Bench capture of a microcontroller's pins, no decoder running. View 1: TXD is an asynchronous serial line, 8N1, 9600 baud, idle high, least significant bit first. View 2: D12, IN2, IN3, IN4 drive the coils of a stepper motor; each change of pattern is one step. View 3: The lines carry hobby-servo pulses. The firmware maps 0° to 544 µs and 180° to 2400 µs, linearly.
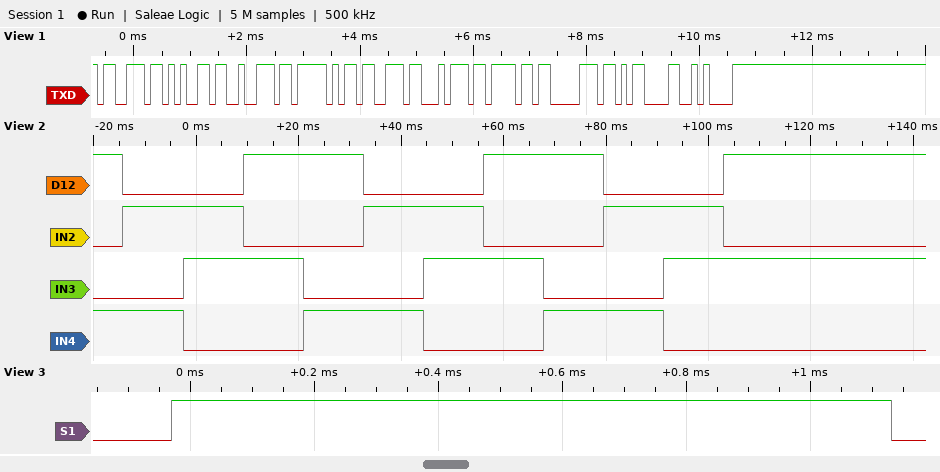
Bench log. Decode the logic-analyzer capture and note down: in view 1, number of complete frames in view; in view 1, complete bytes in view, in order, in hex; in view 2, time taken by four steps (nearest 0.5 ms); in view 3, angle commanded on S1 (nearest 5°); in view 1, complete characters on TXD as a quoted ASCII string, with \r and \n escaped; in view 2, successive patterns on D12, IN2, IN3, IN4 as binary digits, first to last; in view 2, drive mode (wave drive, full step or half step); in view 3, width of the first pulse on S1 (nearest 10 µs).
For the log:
10
73 65 72 5F 73 74 6F 70 0D 0A
47.0 ms
60°
"ser_stop\r\n"
1001 0101 0110 1010 1001 0101 0110 1010 1001 0101 0110 1010
full step
1160 µs
